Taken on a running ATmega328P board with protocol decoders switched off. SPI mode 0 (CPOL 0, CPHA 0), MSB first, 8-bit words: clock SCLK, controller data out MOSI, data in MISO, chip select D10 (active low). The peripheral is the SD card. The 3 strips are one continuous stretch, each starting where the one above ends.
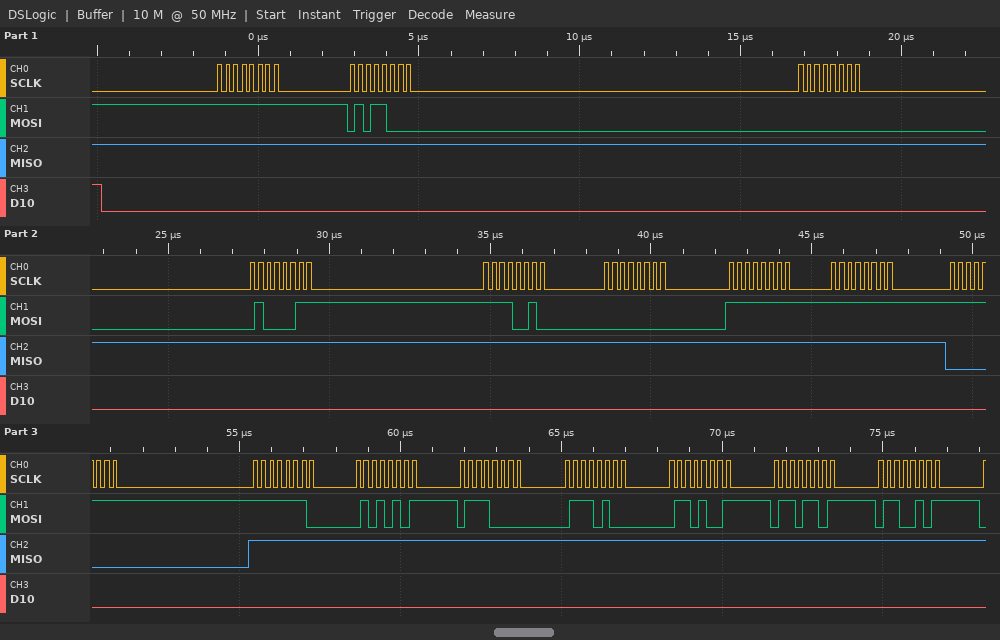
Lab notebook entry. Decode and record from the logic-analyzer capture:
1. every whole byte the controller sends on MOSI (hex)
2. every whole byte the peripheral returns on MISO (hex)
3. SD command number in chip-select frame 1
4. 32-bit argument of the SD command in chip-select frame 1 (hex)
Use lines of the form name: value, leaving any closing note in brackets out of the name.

every whole byte the controller sends on MOSI: FF 58 00 43 F2 00 FF FF FF FE 55 70 74 69 6D 65
every whole byte the peripheral returns on MISO: FF FF FF FF FF FF FF FF 00 FF FF FF FF FF FF FF
SD command number in chip-select frame 1: CMD24
32-bit argument of the SD command in chip-select frame 1: 0x0043F200
